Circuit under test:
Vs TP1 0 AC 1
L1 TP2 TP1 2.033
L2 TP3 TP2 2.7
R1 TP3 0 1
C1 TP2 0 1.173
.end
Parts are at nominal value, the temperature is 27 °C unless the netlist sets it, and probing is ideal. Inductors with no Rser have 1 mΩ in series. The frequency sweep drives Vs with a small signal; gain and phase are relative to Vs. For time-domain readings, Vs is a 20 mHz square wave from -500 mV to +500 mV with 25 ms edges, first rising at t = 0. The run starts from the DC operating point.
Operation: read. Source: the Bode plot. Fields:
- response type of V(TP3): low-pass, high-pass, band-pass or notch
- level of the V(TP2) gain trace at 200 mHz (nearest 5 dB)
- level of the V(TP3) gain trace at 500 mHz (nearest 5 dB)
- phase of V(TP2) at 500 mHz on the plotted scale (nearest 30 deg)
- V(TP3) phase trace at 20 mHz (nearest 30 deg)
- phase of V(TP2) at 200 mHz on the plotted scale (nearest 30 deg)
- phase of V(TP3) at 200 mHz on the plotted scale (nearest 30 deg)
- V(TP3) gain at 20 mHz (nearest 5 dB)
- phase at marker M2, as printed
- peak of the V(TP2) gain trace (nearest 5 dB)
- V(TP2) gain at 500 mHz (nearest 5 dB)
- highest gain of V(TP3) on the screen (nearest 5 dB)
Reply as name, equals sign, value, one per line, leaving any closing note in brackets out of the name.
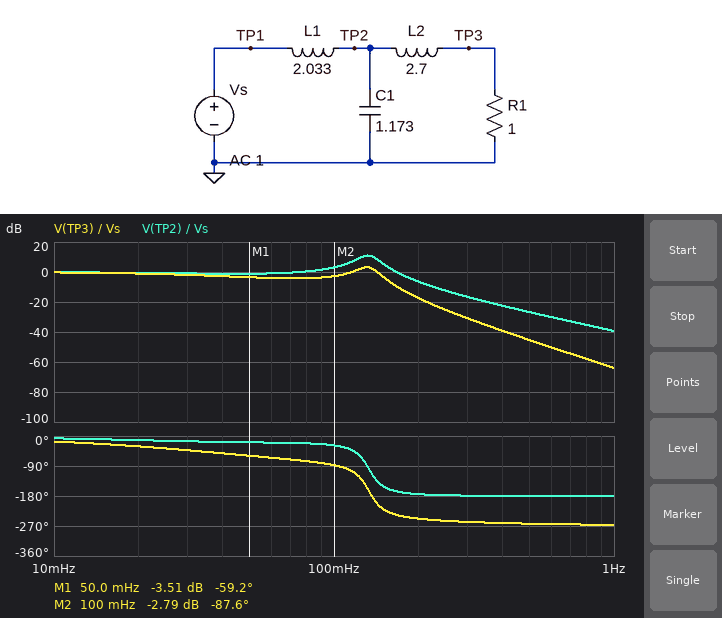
response type of V(TP3): low-pass, high-pass, band-pass or notch = low-pass
level of the V(TP2) gain trace at 200 mHz = -5 dB
level of the V(TP3) gain trace at 500 mHz = -45 dB
phase of V(TP2) at 500 mHz on the plotted scale = -180 deg
V(TP3) phase trace at 20 mHz = -30 deg
phase of V(TP2) at 200 mHz on the plotted scale = -180 deg
phase of V(TP3) at 200 mHz on the plotted scale = -240 deg
V(TP3) gain at 20 mHz = 0 dB
phase at marker M2, as printed = -87.6 deg
peak of the V(TP2) gain trace = 10 dB
V(TP2) gain at 500 mHz = -25 dB
highest gain of V(TP3) on the screen = 5 dB
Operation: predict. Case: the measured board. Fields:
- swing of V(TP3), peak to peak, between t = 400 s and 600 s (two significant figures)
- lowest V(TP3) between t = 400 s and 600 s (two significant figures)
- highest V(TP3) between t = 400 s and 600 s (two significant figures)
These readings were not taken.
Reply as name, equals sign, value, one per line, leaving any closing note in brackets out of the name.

swing of V(TP3), peak to peak, between t = 400 s and 600 s = 1.1 V
lowest V(TP3) between t = 400 s and 600 s = -550 mV
highest V(TP3) between t = 400 s and 600 s = 550 mV
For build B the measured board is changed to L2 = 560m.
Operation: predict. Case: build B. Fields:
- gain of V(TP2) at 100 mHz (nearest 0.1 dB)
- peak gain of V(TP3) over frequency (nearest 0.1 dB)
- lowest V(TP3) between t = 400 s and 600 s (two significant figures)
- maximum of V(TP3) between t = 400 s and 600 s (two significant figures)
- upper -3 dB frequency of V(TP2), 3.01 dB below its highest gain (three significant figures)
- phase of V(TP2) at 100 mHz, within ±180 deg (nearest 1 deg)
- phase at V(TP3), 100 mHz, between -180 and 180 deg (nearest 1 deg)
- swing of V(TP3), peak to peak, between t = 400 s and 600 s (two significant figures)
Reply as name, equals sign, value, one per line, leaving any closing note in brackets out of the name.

gain of V(TP2) at 100 mHz = -1.8 dB
peak gain of V(TP3) over frequency = 0 dB
lowest V(TP3) between t = 400 s and 600 s = -500 mV
maximum of V(TP3) between t = 400 s and 600 s = 500 mV
upper -3 dB frequency of V(TP2), 3.01 dB below its highest gain = 136 mHz
phase of V(TP2) at 100 mHz, within ±180 deg = -68 deg
phase at V(TP3), 100 mHz, between -180 and 180 deg = -87 deg
swing of V(TP3), peak to peak, between t = 400 s and 600 s = 1.0 V
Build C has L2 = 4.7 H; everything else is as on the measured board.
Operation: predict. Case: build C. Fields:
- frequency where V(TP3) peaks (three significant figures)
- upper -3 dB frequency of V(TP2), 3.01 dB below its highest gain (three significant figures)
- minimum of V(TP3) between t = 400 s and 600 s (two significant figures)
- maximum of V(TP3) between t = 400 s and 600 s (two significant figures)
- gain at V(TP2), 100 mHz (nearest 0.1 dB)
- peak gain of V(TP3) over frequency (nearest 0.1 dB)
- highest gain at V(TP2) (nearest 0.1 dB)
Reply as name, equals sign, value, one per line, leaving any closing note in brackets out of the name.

frequency where V(TP3) peaks = 122 mHz
upper -3 dB frequency of V(TP2), 3.01 dB below its highest gain = 127 mHz
minimum of V(TP3) between t = 400 s and 600 s = -530 mV
maximum of V(TP3) between t = 400 s and 600 s = 530 mV
gain at V(TP2), 100 mHz = 6.6 dB
peak gain of V(TP3) over frequency = 7.5 dB
highest gain at V(TP2) = 19.0 dB
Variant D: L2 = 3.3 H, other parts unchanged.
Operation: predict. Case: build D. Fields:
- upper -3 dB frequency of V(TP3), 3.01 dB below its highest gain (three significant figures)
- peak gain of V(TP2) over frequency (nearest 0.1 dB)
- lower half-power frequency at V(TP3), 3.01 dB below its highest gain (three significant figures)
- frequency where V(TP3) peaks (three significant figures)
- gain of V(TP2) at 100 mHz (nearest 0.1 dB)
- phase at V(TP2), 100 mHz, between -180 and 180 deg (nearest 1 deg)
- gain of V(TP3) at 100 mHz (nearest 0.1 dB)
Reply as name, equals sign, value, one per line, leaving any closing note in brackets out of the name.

upper -3 dB frequency of V(TP3), 3.01 dB below its highest gain = 136 mHz
peak gain of V(TP2) over frequency = 13.8 dB
lower half-power frequency at V(TP3), 3.01 dB below its highest gain = 118 mHz
frequency where V(TP3) peaks = 128 mHz
gain of V(TP2) at 100 mHz = 4.3 dB
phase at V(TP2), 100 mHz, between -180 and 180 deg = -23 deg
gain of V(TP3) at 100 mHz = -2.9 dB
